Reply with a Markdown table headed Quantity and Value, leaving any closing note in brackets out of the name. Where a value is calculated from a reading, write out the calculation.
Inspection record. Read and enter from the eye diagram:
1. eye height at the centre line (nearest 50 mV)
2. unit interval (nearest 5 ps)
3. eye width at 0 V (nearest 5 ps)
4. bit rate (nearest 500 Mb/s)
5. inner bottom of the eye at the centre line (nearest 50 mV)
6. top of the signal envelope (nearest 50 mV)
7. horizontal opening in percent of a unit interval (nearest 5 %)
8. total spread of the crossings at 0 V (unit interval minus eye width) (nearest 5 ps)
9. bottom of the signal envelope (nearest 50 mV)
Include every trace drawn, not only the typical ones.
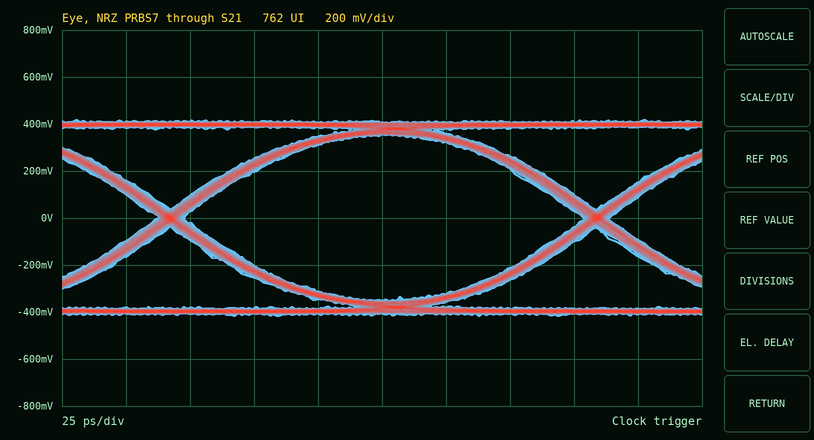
| Quantity | Value |
|---|---|
| eye height at the centre line | 700 mV |
| unit interval | 165 ps |
| eye width at 0 V | 155 ps |
| bit rate | 6.0 Gb/s |
| inner bottom of the eye at the centre line | -350 mV |
| top of the signal envelope | 400 mV |
| horizontal opening in percent of a unit interval | 155 ps / 165 ps ≈ 93.9 %, so 95 % to the nearest 5 % |
| total spread of the crossings at 0 V (unit interval minus eye width) | 10 ps |
| bottom of the signal envelope | -400 mV |
